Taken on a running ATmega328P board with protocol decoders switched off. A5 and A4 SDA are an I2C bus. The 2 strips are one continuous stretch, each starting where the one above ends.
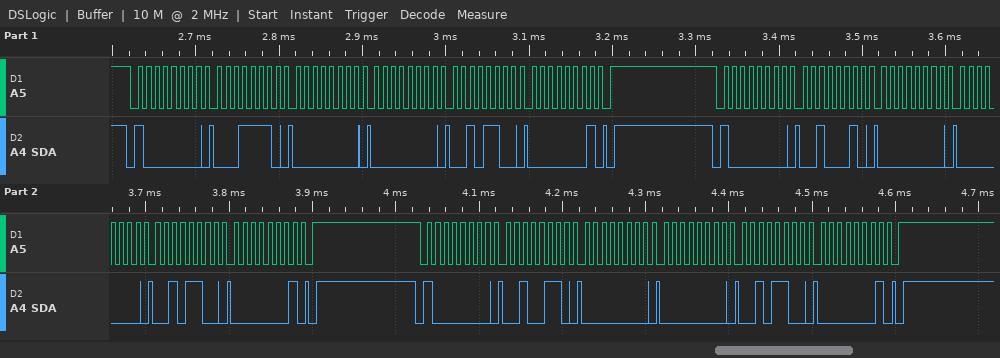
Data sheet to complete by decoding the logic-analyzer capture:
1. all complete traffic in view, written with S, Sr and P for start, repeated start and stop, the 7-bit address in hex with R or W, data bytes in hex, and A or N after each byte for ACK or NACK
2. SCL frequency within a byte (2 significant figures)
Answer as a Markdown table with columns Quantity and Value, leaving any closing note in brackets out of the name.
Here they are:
| Quantity | Value |
|---|---|
| all complete traffic in view, written with S, Sr and P for start, repeated start and stop, the 7-bit address in hex with R or W, data bytes in hex, and A or N after each byte for ACK or NACK | S 40W A 1E A 00 A 00 A 2C A 01 A P S 40W A 22 A 00 A 00 A 2C A 01 A P S 40W A 26 A 00 A 00 A 2C A 01 A P |
| SCL frequency within a byte | 100 kHz |
